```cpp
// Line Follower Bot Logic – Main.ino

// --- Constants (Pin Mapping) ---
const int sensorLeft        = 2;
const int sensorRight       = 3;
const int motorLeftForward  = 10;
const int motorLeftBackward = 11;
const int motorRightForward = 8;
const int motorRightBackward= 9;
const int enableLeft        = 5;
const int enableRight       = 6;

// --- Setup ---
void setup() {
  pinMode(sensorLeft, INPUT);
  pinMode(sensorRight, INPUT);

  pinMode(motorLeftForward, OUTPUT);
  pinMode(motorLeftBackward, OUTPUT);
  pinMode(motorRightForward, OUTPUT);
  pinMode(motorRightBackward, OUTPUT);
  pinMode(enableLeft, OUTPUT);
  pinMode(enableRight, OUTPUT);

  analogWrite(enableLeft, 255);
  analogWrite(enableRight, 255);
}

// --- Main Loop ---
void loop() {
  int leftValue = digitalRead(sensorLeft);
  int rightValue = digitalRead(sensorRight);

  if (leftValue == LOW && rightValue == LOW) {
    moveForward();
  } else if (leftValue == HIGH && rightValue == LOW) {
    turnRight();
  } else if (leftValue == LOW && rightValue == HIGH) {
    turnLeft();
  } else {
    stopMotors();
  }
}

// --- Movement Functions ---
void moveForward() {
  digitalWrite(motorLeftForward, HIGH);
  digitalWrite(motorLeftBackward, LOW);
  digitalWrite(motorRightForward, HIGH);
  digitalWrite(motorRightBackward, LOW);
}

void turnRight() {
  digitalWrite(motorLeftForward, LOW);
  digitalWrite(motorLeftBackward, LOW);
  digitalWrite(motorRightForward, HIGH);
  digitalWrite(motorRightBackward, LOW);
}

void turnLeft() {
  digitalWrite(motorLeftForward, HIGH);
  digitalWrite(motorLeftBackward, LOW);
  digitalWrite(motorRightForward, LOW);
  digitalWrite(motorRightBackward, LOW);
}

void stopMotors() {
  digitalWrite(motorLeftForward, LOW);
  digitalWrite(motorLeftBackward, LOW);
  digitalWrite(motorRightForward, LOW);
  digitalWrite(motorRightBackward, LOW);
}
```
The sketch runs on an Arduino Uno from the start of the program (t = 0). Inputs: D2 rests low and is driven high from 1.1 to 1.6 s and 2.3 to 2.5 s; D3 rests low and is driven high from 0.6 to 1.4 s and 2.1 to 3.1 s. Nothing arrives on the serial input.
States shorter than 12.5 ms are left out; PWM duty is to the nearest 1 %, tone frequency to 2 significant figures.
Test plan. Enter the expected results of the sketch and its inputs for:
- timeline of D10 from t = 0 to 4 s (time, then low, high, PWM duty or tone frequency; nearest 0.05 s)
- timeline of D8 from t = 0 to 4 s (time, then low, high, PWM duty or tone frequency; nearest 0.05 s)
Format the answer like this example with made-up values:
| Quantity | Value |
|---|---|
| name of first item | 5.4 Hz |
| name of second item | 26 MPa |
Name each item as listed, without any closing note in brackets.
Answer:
| Quantity | Value |
|---|---|
| timeline of D10 from t = 0 to 4 s | 0 s high; 1.1 s low; 1.6 s high; 2.3 s low; 2.5 s high |
| timeline of D8 from t = 0 to 4 s | 0 s high; 0.6 s low; 1.4 s high; 2.1 s low; 3.1 s high |
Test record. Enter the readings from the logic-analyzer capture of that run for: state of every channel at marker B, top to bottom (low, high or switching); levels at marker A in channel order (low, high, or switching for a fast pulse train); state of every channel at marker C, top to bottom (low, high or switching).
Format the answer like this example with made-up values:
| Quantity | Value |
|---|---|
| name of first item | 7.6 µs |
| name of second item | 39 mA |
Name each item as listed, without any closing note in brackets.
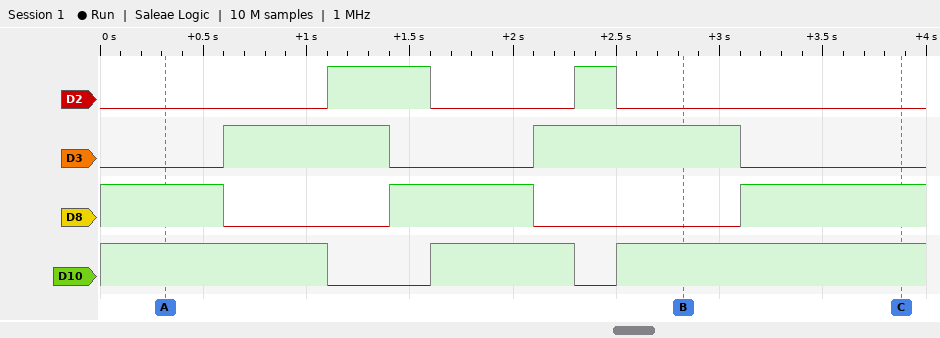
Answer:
| Quantity | Value |
|---|---|
| state of every channel at marker B, top to bottom | D2 low, D3 high, D8 low, D10 high |
| levels at marker A in channel order | D2 low, D3 low, D8 high, D10 high |
| state of every channel at marker C, top to bottom | D2 low, D3 low, D8 high, D10 high |
